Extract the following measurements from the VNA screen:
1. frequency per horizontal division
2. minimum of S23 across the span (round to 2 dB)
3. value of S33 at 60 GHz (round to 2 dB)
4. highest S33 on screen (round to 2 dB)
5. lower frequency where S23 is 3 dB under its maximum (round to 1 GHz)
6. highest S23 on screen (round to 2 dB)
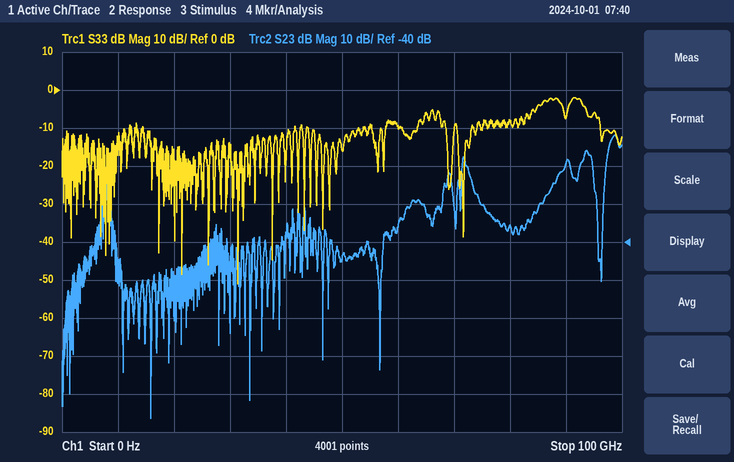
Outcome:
10 GHz
-86 dB
-10 dB
-2 dB
98 GHz
-12 dB
